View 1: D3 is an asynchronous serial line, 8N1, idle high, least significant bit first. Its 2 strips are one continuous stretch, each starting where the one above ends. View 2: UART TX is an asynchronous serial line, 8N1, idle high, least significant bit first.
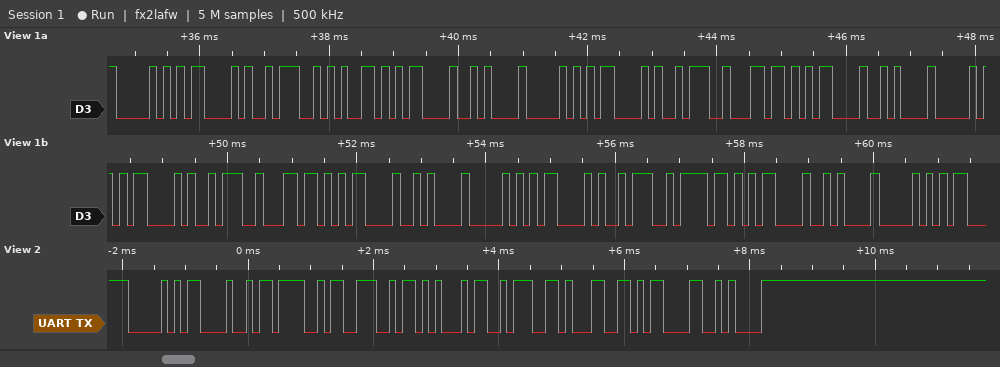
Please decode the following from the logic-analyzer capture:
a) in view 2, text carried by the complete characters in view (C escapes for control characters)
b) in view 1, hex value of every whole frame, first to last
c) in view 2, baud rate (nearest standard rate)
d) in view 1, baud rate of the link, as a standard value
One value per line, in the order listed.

"PHONE:1\r\n"
50 43 3A 65 0D 0A 50 43 3A 6C 0D 0A 50 43 3A 6C 0D 0A 50 43 3A 6F 0D 0A 50
9600 baud
9600 baud
